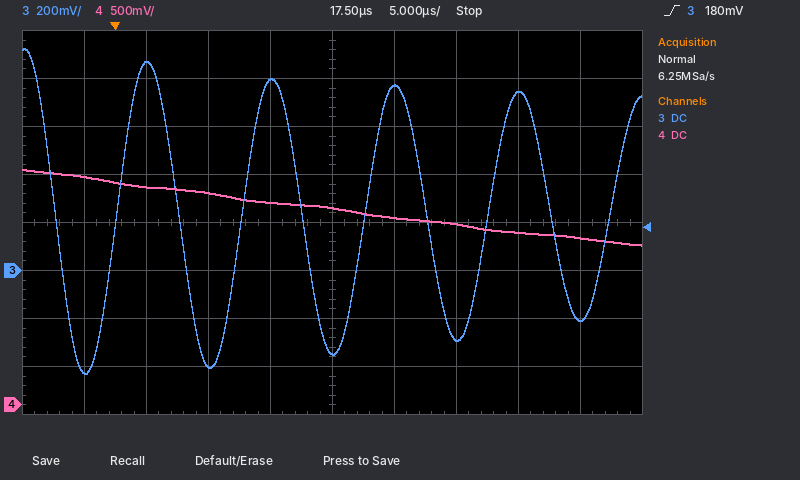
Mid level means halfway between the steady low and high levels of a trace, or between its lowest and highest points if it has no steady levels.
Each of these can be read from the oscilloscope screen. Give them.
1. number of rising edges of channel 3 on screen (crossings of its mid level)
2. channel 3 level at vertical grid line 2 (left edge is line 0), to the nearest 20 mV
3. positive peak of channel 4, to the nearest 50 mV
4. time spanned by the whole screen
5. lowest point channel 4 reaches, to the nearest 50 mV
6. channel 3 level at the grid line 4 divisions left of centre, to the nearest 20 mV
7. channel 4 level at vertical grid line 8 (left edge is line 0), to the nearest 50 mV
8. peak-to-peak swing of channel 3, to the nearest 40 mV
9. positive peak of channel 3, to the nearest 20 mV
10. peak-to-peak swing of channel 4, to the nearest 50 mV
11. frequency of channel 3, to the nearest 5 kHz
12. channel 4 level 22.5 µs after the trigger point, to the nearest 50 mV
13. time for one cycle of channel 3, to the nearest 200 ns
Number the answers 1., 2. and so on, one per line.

1. 5
2. 860 mV
3. 2.45 V
4. 50 µs
5. 1.65 V
6. -420 mV
7. 1.80 V
8. 1.36 V
9. 920 mV
10. 800 mV
11. 100 kHz
12. 1.95 V
13. 10.0 µs
